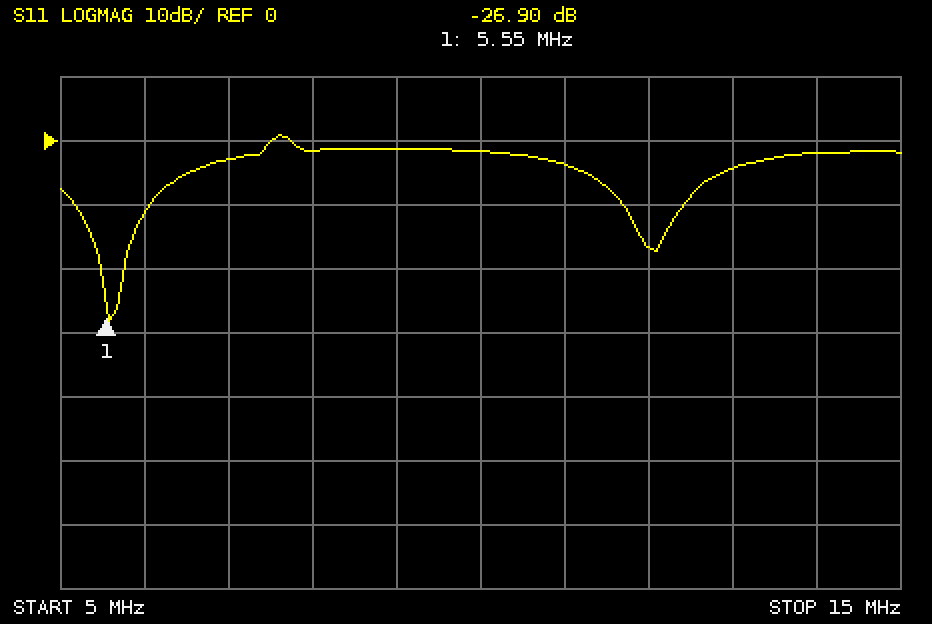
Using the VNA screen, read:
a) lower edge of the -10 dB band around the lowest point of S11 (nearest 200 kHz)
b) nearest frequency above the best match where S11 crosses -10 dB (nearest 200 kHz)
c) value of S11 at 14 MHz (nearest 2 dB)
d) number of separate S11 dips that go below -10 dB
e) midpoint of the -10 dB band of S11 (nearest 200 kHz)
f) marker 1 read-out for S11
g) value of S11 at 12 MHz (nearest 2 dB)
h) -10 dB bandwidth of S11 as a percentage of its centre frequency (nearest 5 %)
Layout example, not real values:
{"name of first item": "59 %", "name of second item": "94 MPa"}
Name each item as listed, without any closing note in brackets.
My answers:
{"lower edge of the -10 dB band around the lowest point of S11": "5.2 MHz", "nearest frequency above the best match where S11 crosses -10 dB": "6.0 MHz", "value of S11 at 14 MHz": "-2 dB", "number of separate S11 dips that go below -10 dB": "2", "midpoint of the -10 dB band of S11": "5.6 MHz", "marker 1 read-out for S11": "-26.90 dB", "value of S11 at 12 MHz": "-16 dB", "-10 dB bandwidth of S11 as a percentage of its centre frequency": "15 %"}
